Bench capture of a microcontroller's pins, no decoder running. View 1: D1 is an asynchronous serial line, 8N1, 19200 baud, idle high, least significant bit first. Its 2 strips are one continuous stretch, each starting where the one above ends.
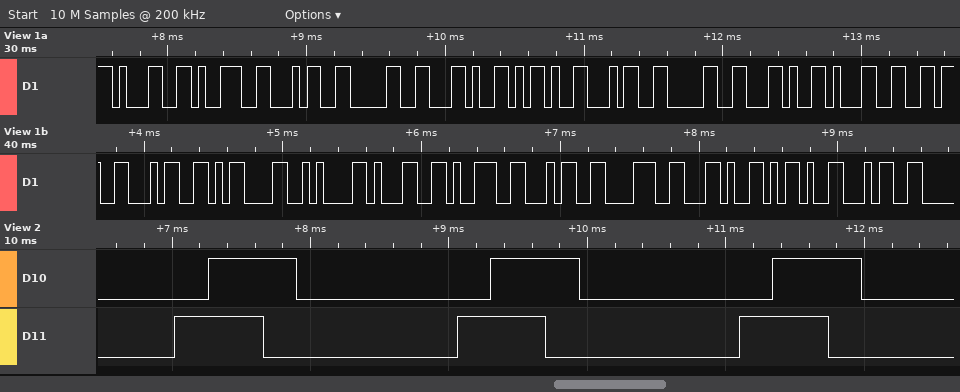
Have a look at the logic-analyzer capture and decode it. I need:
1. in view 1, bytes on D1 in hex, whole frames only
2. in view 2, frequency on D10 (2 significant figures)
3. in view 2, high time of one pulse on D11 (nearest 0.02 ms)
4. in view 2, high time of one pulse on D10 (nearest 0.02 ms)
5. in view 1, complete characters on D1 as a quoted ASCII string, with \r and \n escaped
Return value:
31 39 34 30 2C 2D 34 30 2C 31 36 34 0D 0A 31 39 34 38 2C 2D 34
490 Hz
0.64 ms
0.64 ms
"1940,-40,164\r\n1948,-4"
